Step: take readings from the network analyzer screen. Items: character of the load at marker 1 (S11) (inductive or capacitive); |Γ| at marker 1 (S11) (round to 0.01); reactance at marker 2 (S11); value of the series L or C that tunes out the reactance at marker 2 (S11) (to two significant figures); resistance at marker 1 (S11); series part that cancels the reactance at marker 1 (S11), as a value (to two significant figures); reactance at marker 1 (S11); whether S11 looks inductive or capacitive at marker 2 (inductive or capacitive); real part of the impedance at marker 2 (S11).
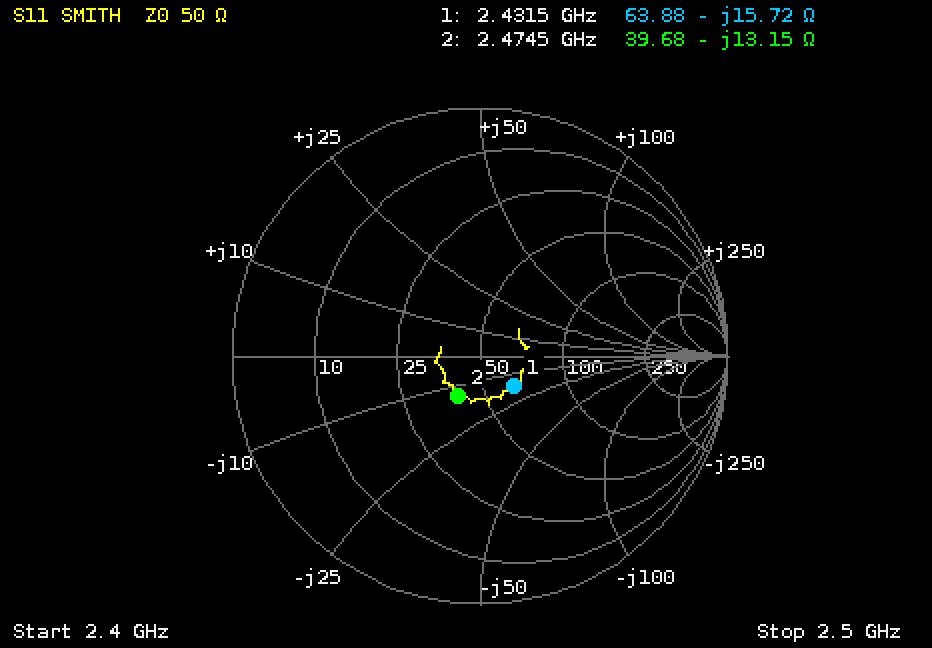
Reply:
capacitive
0.18
-13.15 Ω
850 pH
63.88 Ω
1.0 nH
-15.72 Ω
capacitive
39.68 Ω
